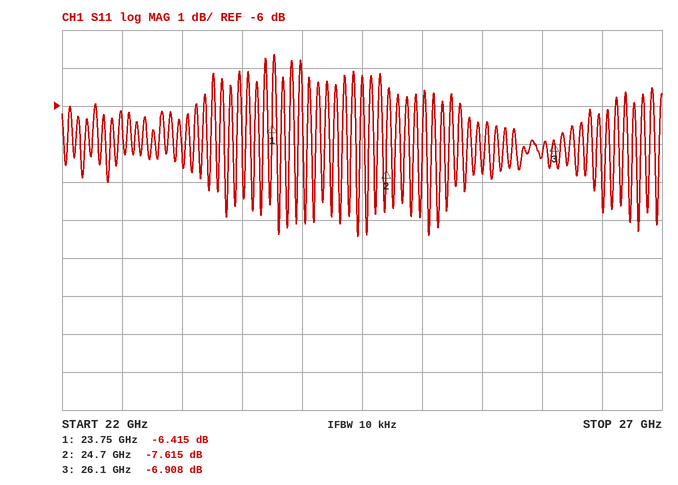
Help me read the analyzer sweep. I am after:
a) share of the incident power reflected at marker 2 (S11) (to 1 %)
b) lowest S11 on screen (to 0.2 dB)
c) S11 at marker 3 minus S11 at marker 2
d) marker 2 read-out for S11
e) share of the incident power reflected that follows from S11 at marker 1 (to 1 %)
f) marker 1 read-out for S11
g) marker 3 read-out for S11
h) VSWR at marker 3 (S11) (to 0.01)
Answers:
17 %
-9.4 dB
0.707 dB
-7.615 dB
23 %
-6.415 dB
-6.908 dB
2.65
